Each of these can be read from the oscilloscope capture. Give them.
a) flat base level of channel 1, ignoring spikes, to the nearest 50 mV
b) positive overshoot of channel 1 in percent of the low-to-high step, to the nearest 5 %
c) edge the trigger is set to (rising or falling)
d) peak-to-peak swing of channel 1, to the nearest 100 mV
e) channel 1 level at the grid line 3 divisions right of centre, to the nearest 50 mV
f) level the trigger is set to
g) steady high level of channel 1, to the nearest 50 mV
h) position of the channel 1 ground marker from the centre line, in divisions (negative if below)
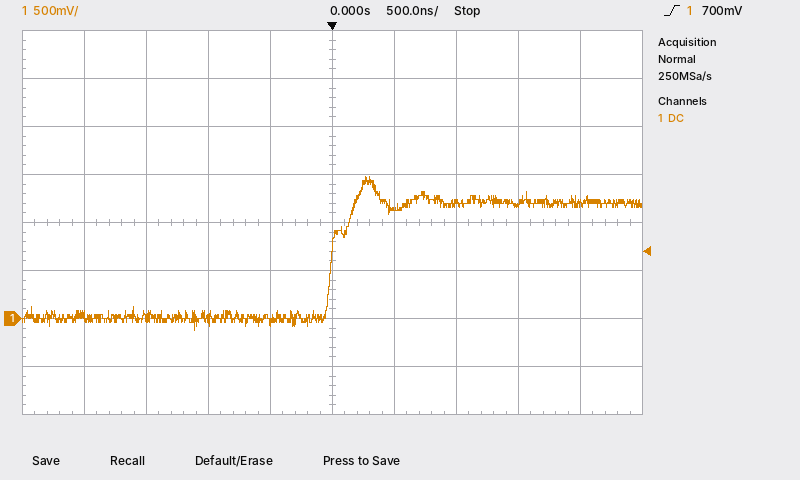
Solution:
0 mV
20 %
rising
1.60 V
1.20 V
700 mV
1.20 V
-2.0 div
